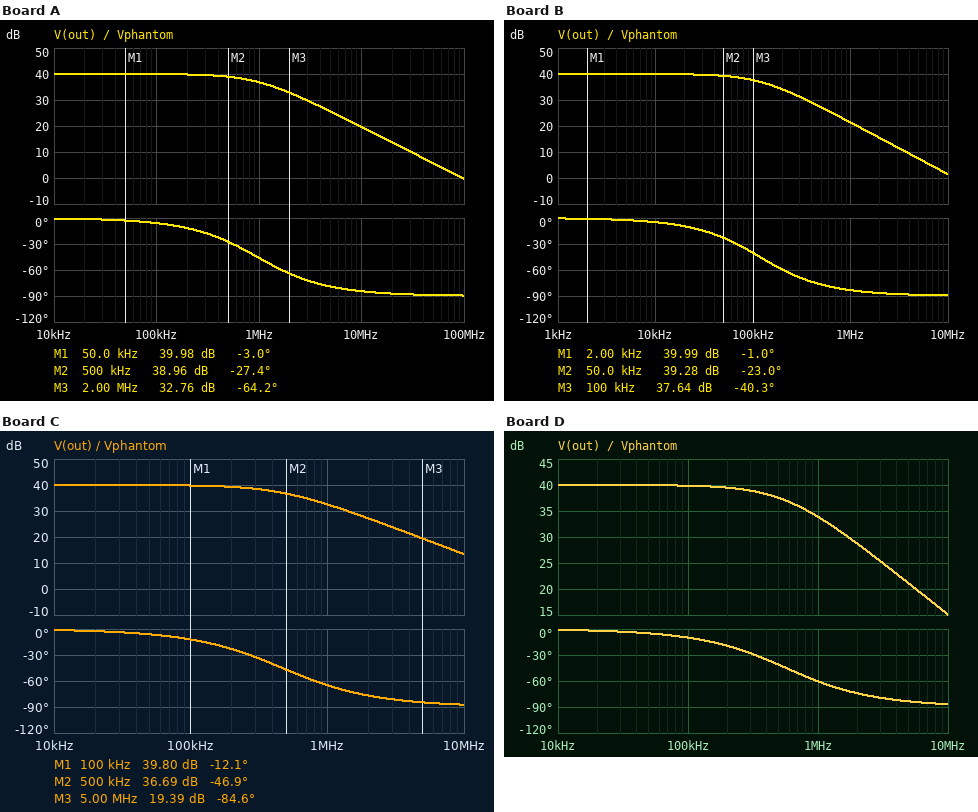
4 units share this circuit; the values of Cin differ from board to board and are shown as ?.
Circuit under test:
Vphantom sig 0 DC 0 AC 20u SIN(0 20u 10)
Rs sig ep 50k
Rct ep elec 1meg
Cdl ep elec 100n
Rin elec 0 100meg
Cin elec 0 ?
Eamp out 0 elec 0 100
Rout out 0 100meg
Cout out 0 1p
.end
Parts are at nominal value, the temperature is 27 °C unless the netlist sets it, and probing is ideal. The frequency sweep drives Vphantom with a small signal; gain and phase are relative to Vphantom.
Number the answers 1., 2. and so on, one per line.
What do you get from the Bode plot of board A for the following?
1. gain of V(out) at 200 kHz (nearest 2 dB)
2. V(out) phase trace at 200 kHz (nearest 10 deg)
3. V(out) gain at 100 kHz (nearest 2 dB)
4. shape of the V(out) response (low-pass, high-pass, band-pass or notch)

1. 40 dB
2. -10 deg
3. 40 dB
4. low-pass
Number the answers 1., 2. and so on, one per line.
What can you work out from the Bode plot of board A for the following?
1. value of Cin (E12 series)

1. 3.3 pF
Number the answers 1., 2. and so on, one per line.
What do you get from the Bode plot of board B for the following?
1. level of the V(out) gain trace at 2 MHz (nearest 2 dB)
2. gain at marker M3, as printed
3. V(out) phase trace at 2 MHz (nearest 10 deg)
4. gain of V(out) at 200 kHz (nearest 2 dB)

1. 16 dB
2. 37.64 dB
3. -90 deg
4. 34 dB
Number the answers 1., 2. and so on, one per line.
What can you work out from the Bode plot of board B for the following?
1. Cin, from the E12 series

1. 27 pF
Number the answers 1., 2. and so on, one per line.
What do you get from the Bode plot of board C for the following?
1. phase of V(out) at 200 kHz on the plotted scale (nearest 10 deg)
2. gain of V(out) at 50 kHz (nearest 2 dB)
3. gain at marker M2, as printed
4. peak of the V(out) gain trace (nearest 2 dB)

1. -20 deg
2. 40 dB
3. 36.69 dB
4. 40 dB
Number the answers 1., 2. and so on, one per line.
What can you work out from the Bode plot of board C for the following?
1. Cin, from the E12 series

1. 6.8 pF
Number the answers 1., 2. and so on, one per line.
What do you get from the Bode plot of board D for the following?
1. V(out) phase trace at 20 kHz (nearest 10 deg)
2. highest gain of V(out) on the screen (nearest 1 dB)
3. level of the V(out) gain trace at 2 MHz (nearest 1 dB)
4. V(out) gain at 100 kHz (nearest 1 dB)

1. 0 deg
2. 40 dB
3. 29 dB
4. 40 dB
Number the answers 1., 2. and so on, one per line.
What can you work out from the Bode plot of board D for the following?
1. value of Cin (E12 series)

1. 5.6 pF
